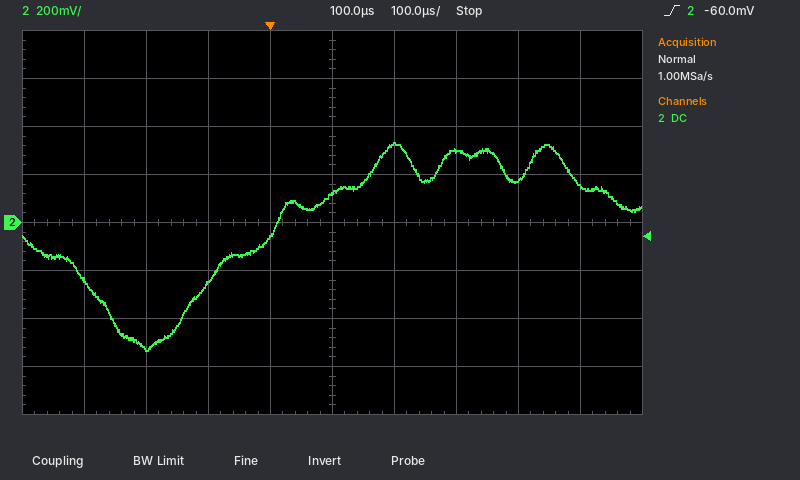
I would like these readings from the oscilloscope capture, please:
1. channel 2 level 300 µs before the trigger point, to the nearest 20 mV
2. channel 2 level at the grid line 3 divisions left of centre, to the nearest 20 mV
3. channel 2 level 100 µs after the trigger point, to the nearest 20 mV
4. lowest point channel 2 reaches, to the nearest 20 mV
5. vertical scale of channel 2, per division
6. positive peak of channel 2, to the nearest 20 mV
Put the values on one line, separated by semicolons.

-240 mV; -520 mV; 120 mV; -540 mV; 200 mV; 340 mV
